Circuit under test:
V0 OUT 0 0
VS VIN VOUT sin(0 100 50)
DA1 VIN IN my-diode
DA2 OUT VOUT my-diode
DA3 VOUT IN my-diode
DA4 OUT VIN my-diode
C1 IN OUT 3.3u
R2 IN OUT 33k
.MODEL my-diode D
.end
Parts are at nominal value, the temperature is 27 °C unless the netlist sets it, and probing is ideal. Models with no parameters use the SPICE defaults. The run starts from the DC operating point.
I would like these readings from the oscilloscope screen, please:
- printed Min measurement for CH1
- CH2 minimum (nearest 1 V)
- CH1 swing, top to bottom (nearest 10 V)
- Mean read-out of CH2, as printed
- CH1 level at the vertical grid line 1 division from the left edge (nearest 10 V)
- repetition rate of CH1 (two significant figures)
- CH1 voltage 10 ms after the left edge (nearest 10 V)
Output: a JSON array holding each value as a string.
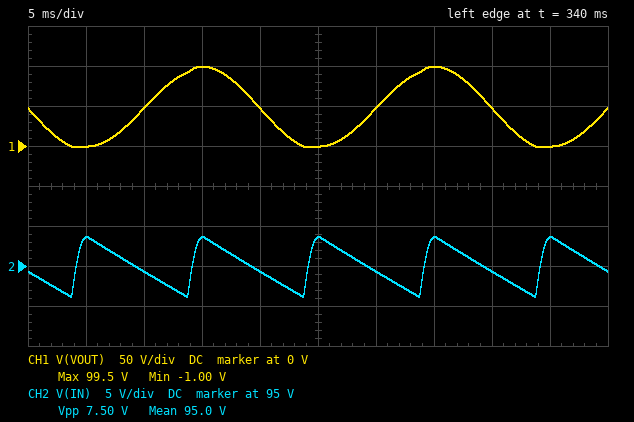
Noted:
["-1.00 V", "91 V", "100 V", "95.0 V", "0 V", "50 Hz", "50 V"]
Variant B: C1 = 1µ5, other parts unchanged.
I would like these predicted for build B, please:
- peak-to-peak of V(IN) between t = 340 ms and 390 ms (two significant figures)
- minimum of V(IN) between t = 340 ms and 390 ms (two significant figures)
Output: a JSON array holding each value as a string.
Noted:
["15 V", "84 V"]
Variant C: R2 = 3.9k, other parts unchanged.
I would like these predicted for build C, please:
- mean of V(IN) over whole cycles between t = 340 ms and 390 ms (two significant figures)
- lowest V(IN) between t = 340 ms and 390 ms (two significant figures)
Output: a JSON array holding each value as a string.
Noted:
["80 V", "59 V"]
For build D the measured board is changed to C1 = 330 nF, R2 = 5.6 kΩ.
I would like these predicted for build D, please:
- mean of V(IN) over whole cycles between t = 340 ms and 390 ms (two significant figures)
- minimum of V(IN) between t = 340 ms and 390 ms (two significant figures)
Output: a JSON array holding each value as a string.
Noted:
["64 V", "15 V"]
